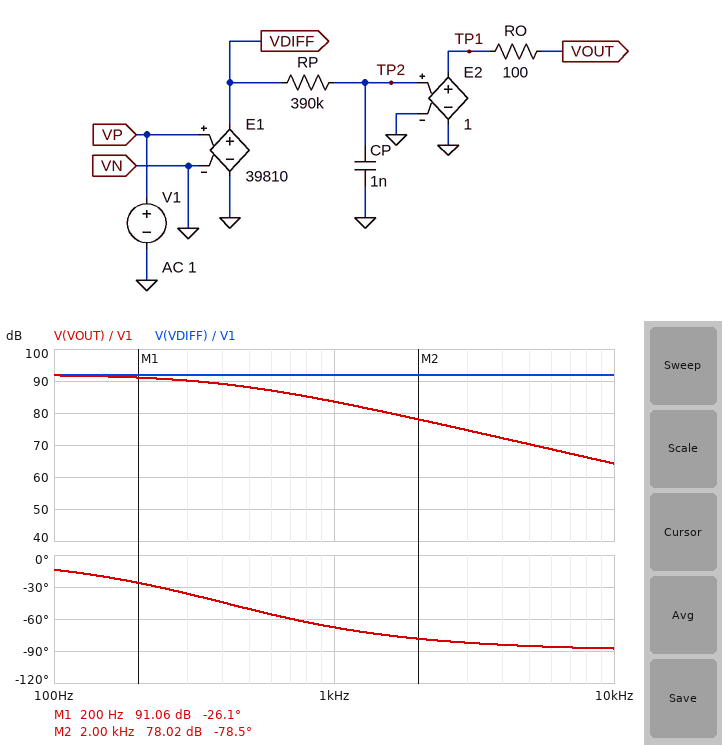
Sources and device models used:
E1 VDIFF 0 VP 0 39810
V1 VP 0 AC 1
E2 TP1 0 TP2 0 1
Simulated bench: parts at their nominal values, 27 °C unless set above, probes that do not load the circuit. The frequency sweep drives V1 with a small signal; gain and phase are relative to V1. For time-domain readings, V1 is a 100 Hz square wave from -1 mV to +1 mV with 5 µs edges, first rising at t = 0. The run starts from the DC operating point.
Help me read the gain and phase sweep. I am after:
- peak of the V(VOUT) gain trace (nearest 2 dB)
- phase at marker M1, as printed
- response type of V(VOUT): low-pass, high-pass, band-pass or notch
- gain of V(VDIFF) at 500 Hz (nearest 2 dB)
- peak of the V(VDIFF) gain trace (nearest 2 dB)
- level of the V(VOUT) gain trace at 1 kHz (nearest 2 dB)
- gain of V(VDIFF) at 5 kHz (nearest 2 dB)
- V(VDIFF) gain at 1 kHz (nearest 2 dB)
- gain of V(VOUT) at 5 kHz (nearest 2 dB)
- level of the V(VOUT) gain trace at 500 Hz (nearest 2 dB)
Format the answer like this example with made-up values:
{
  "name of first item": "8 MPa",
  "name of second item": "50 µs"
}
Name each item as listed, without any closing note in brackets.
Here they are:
{
  "peak of the V(VOUT) gain trace": "92 dB",
  "phase at marker M1, as printed": "-26.1 deg",
  "response type of V(VOUT): low-pass, high-pass, band-pass or notch": "low-pass",
  "gain of V(VDIFF) at 500 Hz": "92 dB",
  "peak of the V(VDIFF) gain trace": "92 dB",
  "level of the V(VOUT) gain trace at 1 kHz": "84 dB",
  "gain of V(VDIFF) at 5 kHz": "92 dB",
  "V(VDIFF) gain at 1 kHz": "92 dB",
  "gain of V(VOUT) at 5 kHz": "70 dB",
  "level of the V(VOUT) gain trace at 500 Hz": "88 dB"
}
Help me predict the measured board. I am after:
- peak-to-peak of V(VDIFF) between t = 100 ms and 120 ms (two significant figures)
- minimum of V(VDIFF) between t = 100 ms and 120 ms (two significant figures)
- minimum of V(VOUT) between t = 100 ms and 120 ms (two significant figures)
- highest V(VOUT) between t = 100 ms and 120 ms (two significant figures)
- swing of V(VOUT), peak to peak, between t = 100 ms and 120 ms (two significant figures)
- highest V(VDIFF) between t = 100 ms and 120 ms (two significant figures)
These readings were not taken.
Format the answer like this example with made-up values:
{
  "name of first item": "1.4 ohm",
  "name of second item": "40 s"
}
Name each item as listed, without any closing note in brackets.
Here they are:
{
  "peak-to-peak of V(VDIFF) between t = 100 ms and 120 ms": "80 V",
  "minimum of V(VDIFF) between t = 100 ms and 120 ms": "-40 V",
  "minimum of V(VOUT) between t = 100 ms and 120 ms": "-40 V",
  "highest V(VOUT) between t = 100 ms and 120 ms": "40 V",
  "swing of V(VOUT), peak to peak, between t = 100 ms and 120 ms": "80 V",
  "highest V(VDIFF) between t = 100 ms and 120 ms": "40 V"
}
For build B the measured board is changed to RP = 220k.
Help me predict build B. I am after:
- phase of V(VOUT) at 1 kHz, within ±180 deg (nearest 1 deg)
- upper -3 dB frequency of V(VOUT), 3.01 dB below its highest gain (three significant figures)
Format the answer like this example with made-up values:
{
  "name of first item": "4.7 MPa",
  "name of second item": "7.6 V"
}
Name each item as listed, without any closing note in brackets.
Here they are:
{
  "phase of V(VOUT) at 1 kHz, within ±180 deg": "-54 deg",
  "upper -3 dB frequency of V(VOUT), 3.01 dB below its highest gain": "723 Hz"
}
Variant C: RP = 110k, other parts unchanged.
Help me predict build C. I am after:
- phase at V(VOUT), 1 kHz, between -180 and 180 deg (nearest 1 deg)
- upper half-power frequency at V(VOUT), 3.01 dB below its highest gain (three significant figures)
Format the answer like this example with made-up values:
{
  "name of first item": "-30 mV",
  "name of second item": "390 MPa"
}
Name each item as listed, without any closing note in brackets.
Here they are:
{
  "phase at V(VOUT), 1 kHz, between -180 and 180 deg": "-35 deg",
  "upper half-power frequency at V(VOUT), 3.01 dB below its highest gain": "1.45 kHz"
}
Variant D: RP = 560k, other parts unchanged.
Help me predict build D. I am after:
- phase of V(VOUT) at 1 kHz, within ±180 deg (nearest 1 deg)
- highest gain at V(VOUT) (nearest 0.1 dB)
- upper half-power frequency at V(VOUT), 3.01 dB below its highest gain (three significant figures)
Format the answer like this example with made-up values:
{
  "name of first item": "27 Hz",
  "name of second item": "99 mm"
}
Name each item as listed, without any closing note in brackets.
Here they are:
{
  "phase of V(VOUT) at 1 kHz, within ±180 deg": "-74 deg",
  "highest gain at V(VOUT)": "92.0 dB",
  "upper half-power frequency at V(VOUT), 3.01 dB below its highest gain": "284 Hz"
}
